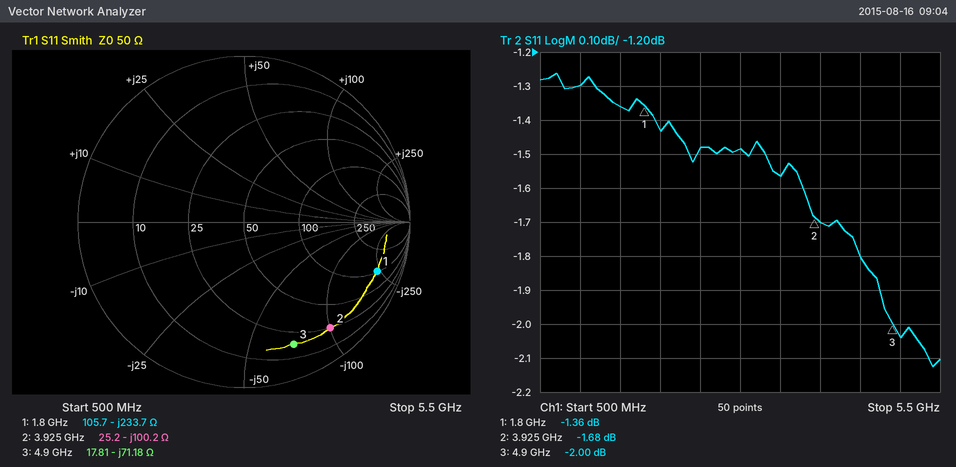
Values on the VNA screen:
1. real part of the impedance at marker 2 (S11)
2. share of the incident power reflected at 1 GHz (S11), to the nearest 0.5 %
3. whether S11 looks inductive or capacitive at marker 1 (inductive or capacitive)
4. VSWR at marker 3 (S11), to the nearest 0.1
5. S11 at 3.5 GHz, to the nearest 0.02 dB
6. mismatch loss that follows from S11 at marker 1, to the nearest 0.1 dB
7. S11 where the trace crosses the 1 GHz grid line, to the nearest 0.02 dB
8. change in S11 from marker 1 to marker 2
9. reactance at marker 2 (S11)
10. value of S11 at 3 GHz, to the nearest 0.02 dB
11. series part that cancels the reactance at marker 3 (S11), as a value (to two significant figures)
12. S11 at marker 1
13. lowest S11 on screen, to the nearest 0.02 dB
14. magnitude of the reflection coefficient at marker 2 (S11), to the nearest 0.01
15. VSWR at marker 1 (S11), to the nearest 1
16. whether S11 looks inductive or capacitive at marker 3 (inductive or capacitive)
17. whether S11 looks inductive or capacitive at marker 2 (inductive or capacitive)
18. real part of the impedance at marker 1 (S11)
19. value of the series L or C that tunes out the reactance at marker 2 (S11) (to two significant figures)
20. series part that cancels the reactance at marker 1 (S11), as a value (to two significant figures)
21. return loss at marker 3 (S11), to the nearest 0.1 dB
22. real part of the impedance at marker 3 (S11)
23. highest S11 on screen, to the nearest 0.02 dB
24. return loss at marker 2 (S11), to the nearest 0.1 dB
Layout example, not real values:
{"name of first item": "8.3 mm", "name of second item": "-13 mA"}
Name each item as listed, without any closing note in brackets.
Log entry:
{"real part of the impedance at marker 2": "25.2 Ω", "share of the incident power reflected at 1 GHz (S11), to the nearest 0.5 %": "74.0 %", "whether S11 looks inductive or capacitive at marker 1": "capacitive", "VSWR at marker 3 (S11), to the nearest 0.1": "8.7", "S11 at 3.5 GHz, to the nearest 0.02 dB": "-1.56 dB", "mismatch loss that follows from S11 at marker 1, to the nearest 0.1 dB": "5.7 dB", "S11 where the trace crosses the 1 GHz grid line, to the nearest 0.02 dB": "-1.30 dB", "change in S11 from marker 1 to marker 2": "-0.32 dB", "reactance at marker 2": "-100.2 Ω", "value of S11 at 3 GHz, to the nearest 0.02 dB": "-1.48 dB", "series part that cancels the reactance at marker 3 (S11), as a value": "2.3 nH", "S11 at marker 1": "-1.36 dB", "lowest S11 on screen, to the nearest 0.02 dB": "-2.12 dB", "magnitude of the reflection coefficient at marker 2 (S11), to the nearest 0.01": "0.82", "VSWR at marker 1 (S11), to the nearest 1": "13", "whether S11 looks inductive or capacitive at marker 3": "capacitive", "whether S11 looks inductive or capacitive at marker 2": "capacitive", "real part of the impedance at marker 1": "105.7 Ω", "value of the series L or C that tunes out the reactance at marker 2 (S11)": "4.1 nH", "series part that cancels the reactance at marker 1 (S11), as a value": "21 nH", "return loss at marker 3 (S11), to the nearest 0.1 dB": "2.0 dB", "real part of the impedance at marker 3": "17.81 Ω", "highest S11 on screen, to the nearest 0.02 dB": "-1.26 dB", "return loss at marker 2 (S11), to the nearest 0.1 dB": "1.7 dB"}
